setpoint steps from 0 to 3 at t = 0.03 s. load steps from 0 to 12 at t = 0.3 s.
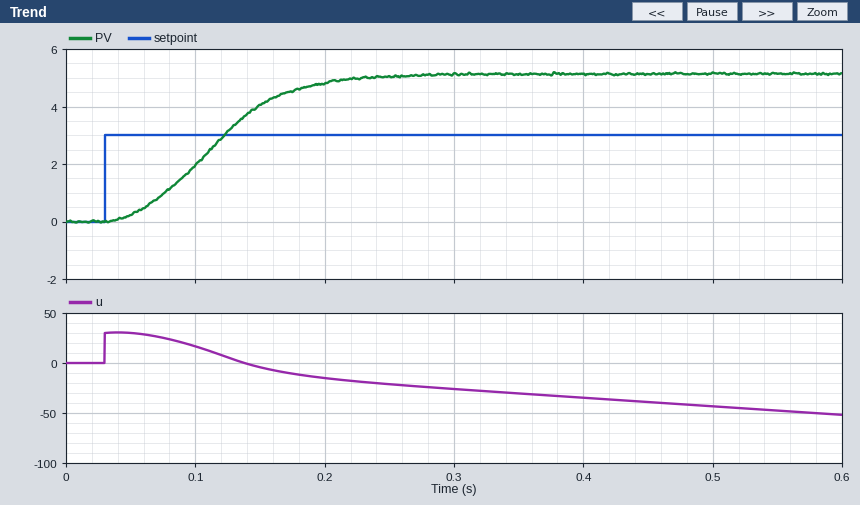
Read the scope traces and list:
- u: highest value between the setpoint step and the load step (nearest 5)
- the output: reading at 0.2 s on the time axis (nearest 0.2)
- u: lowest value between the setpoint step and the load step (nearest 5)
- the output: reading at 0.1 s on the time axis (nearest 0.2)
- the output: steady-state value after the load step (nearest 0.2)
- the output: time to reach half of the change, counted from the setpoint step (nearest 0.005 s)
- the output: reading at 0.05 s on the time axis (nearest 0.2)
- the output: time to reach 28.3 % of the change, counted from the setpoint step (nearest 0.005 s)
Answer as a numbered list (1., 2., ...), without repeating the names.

1. 30
2. 4.8
3. -25
4. 2.0
5. 5.2
6. 0.085 s
7. 0.2
8. 0.060 s
